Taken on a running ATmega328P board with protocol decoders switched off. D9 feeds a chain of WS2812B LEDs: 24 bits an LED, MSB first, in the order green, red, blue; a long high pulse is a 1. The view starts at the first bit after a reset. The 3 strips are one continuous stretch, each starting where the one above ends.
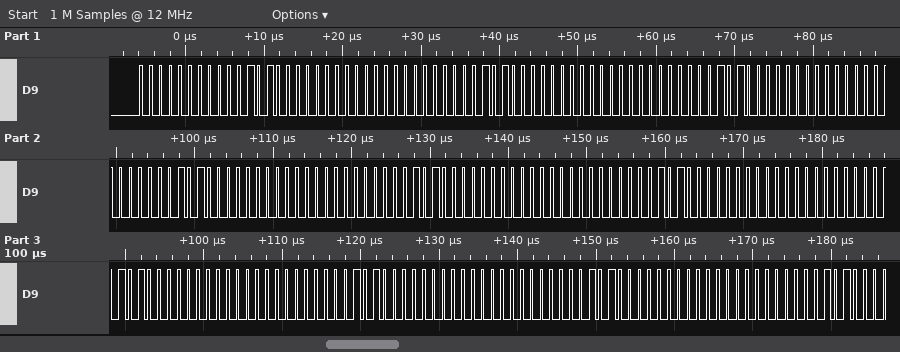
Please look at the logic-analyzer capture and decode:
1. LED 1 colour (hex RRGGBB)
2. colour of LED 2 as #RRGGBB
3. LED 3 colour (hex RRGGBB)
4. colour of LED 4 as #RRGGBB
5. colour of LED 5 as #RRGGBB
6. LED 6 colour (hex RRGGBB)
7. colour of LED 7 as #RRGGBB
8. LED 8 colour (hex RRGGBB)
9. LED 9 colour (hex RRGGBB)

#140000
#140000
#140000
#140000
#140000
#0A0000
#0A0000
#0A0000
#0A0000
